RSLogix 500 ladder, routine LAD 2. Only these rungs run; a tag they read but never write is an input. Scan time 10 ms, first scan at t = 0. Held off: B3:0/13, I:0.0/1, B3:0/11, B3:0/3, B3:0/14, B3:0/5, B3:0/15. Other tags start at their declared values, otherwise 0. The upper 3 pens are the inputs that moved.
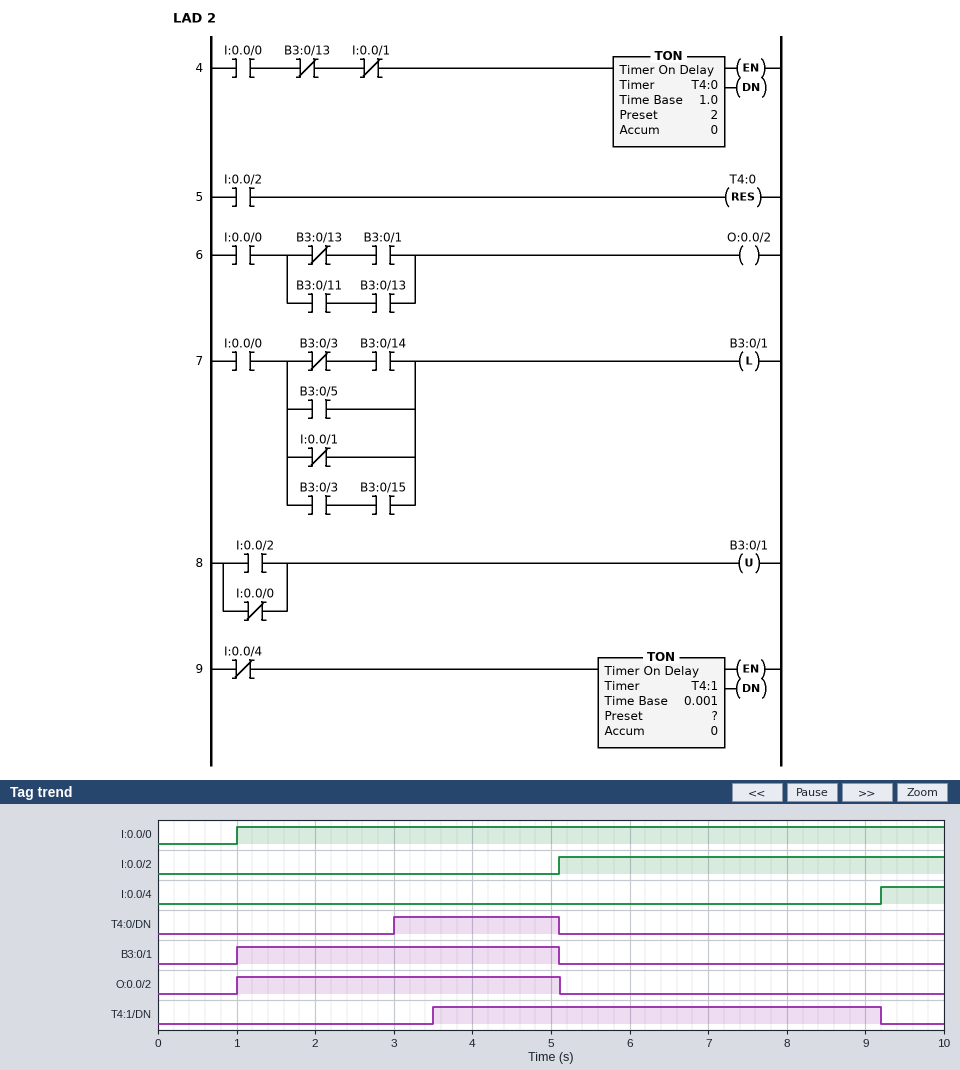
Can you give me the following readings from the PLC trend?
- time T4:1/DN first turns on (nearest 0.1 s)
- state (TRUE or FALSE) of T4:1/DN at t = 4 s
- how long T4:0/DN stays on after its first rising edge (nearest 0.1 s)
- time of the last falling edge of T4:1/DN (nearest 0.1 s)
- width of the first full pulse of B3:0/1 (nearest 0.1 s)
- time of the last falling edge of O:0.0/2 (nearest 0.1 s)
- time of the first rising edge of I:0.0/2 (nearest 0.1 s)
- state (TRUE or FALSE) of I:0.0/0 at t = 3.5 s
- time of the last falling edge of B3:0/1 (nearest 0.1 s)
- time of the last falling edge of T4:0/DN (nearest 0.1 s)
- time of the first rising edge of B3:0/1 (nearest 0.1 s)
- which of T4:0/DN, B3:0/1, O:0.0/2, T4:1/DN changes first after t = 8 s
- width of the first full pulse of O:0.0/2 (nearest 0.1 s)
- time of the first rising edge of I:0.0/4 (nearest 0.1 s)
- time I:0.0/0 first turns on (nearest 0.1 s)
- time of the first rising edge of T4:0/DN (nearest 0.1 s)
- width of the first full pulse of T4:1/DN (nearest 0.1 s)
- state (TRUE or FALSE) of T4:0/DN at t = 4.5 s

3.5 s
TRUE
2.1 s
9.2 s
4.1 s
5.1 s
5.1 s
TRUE
5.1 s
5.1 s
1.0 s
T4:1/DN
4.1 s
9.2 s
1.0 s
3.0 s
5.7 s
TRUE
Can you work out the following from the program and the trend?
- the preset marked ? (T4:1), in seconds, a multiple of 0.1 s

3.5 s
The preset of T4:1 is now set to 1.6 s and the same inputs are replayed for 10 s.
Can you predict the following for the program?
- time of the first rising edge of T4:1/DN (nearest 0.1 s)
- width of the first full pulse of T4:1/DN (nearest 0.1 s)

1.6 s
7.6 s
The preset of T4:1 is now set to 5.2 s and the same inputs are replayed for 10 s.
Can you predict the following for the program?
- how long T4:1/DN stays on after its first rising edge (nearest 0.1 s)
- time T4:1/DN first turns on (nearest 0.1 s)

4.0 s
5.2 s
